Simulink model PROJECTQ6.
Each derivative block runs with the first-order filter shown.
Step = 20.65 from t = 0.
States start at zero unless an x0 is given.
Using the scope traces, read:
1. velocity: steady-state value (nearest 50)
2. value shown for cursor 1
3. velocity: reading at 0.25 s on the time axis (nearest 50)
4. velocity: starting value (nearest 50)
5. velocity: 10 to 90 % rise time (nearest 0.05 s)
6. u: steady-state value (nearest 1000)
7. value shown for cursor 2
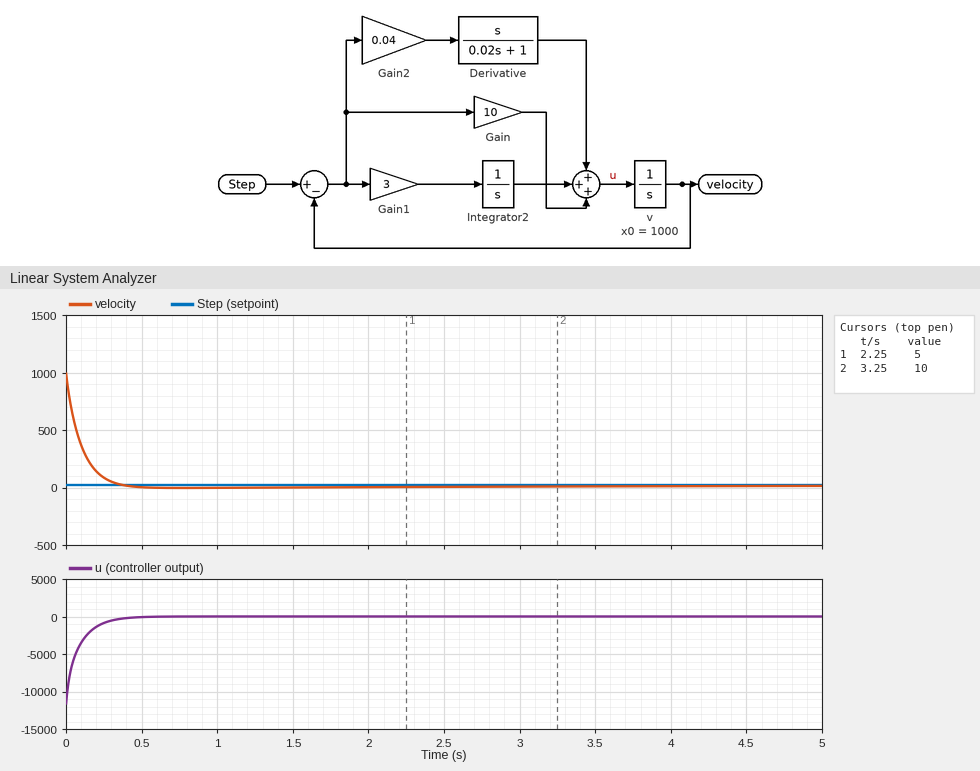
0
5
100
1000
0.20 s
0
10
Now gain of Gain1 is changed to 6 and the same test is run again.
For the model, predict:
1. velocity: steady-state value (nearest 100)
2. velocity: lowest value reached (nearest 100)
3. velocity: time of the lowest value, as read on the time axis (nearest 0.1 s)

0
0
0.6 s
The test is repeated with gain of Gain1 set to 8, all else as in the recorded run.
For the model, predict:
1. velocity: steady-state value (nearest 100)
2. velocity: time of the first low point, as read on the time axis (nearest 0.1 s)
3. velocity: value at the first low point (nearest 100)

0
0.6 s
0
